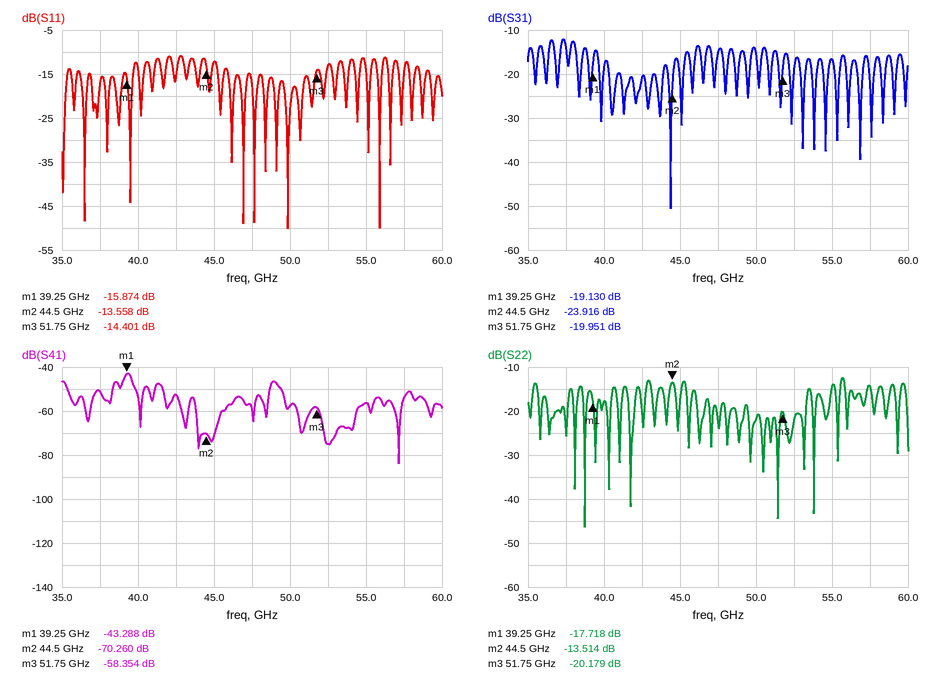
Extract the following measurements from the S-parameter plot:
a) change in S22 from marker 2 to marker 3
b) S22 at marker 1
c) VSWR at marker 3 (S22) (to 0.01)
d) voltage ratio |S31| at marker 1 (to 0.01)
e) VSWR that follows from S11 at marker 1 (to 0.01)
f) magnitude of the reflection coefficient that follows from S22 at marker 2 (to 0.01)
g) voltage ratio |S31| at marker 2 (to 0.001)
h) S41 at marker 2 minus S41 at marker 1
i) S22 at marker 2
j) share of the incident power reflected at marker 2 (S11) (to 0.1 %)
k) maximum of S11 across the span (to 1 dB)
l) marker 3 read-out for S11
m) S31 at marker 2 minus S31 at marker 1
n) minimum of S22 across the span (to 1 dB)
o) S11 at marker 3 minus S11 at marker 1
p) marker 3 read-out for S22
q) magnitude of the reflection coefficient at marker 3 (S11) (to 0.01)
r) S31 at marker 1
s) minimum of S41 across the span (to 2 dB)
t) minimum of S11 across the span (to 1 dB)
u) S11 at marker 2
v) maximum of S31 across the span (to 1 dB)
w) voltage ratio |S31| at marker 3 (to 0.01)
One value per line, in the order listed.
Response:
-6.665 dB
-17.718 dB
1.22
0.11
1.38
0.21
0.064
-26.972 dB
-13.514 dB
4.4 %
-11 dB
-14.401 dB
-4.786 dB
-46 dB
1.473 dB
-20.179 dB
0.19
-19.130 dB
-84 dB
-50 dB
-13.558 dB
-12 dB
0.10
